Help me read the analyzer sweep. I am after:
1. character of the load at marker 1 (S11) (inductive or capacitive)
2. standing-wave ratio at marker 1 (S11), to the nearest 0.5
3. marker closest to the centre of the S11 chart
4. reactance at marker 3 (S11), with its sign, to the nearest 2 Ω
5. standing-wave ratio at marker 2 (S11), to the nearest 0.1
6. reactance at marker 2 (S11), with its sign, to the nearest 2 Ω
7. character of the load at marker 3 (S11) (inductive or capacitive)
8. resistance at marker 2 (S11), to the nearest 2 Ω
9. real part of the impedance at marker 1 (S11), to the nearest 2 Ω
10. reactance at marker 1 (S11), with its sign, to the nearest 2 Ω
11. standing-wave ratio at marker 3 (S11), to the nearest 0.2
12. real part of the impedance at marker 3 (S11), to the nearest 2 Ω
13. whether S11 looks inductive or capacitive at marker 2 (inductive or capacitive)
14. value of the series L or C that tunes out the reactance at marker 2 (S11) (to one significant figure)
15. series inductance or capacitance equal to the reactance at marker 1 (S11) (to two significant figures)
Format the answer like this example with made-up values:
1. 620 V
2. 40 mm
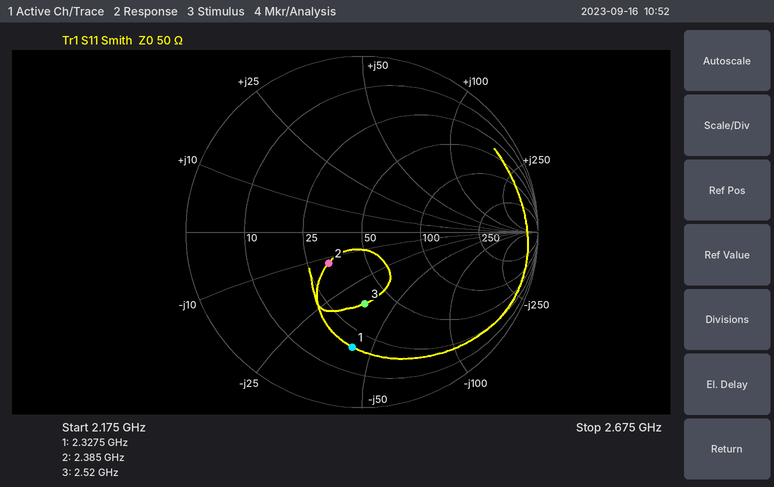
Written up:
1. capacitive
2. 5.0
3. marker 2
4. -36 Ω
5. 1.7
6. -12 Ω
7. capacitive
8. 32 Ω
9. 18 Ω
10. -42 Ω
11. 2.4
12. 36 Ω
13. capacitive
14. 800 pH
15. 1.6 pF
